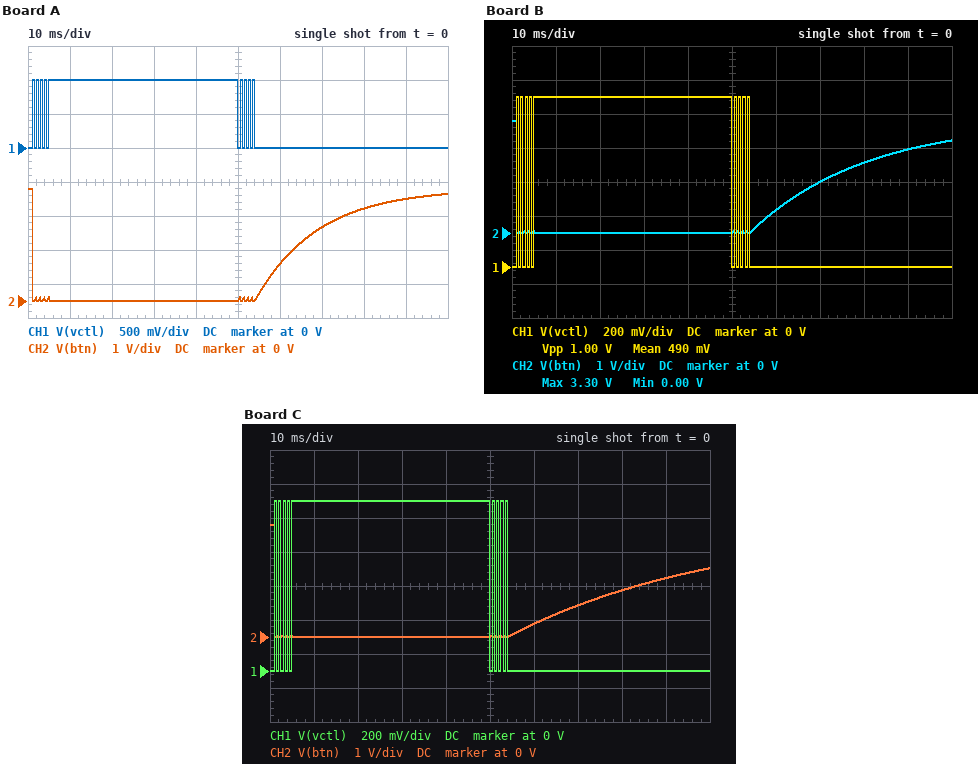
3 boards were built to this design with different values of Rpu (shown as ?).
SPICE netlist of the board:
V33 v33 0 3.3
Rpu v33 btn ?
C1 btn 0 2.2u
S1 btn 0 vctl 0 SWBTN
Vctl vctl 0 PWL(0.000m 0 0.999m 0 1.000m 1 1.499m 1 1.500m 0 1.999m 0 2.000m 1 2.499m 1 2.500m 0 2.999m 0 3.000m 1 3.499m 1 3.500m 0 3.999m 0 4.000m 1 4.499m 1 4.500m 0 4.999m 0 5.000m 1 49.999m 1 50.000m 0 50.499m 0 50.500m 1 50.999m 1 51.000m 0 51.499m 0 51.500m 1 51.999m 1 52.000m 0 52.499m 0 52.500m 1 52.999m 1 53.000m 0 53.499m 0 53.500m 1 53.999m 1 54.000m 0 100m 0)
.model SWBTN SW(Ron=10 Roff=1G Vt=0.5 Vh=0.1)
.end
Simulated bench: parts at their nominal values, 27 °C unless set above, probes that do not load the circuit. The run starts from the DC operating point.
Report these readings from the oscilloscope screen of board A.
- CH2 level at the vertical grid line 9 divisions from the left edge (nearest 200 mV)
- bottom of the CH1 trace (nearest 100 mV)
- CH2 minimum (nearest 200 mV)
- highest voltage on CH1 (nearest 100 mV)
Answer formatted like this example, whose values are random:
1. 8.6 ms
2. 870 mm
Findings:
1. 3.0 V
2. 0 V
3. 0 V
4. 1.0 V
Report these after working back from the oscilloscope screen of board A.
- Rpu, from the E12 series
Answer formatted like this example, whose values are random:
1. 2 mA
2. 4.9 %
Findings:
1. 6.8 kΩ
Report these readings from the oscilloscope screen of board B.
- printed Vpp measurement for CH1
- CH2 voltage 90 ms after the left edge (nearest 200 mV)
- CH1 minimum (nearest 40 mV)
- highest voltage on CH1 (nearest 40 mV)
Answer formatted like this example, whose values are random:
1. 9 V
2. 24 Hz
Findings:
1. 1.00 V
2. 2.4 V
3. 0 V
4. 1.00 V
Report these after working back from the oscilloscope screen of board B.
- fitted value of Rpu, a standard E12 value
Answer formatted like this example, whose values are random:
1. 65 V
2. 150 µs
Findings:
1. 12 kΩ
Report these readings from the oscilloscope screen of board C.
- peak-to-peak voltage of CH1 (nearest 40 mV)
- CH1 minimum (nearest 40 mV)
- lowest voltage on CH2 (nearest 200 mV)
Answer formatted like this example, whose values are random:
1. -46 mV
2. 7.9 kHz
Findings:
1. 1.00 V
2. 0 V
3. 0 V
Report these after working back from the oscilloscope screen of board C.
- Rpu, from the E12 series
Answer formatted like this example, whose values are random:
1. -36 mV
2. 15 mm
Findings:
1. 22 kΩ
